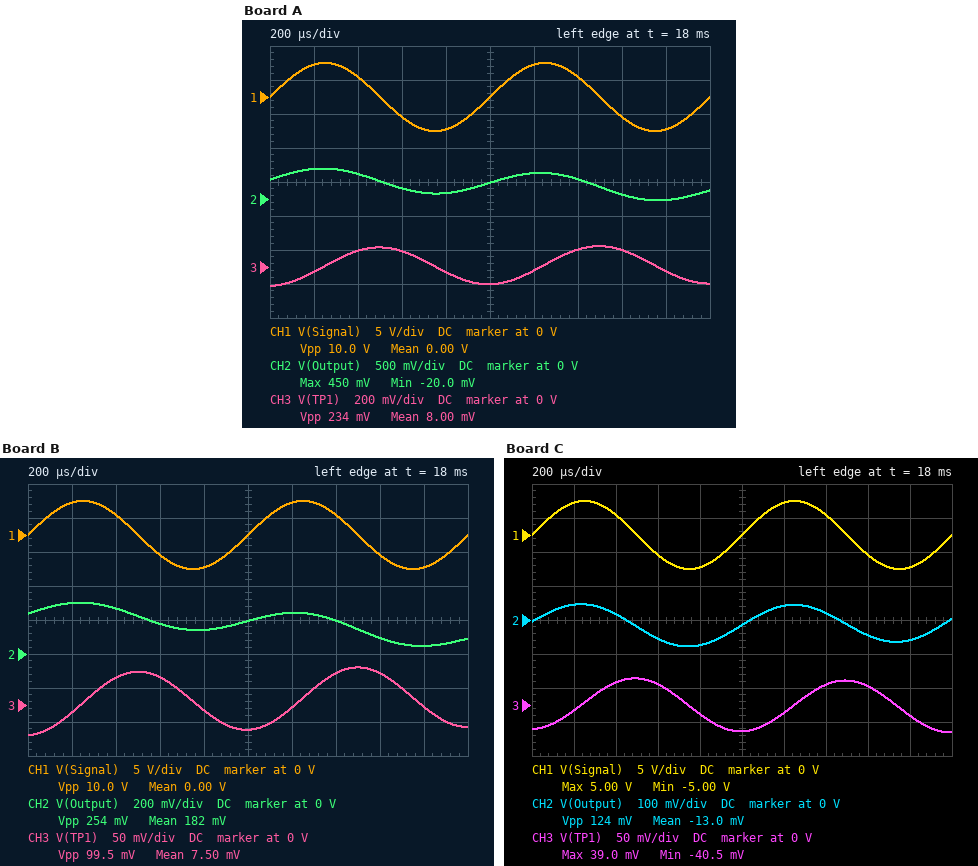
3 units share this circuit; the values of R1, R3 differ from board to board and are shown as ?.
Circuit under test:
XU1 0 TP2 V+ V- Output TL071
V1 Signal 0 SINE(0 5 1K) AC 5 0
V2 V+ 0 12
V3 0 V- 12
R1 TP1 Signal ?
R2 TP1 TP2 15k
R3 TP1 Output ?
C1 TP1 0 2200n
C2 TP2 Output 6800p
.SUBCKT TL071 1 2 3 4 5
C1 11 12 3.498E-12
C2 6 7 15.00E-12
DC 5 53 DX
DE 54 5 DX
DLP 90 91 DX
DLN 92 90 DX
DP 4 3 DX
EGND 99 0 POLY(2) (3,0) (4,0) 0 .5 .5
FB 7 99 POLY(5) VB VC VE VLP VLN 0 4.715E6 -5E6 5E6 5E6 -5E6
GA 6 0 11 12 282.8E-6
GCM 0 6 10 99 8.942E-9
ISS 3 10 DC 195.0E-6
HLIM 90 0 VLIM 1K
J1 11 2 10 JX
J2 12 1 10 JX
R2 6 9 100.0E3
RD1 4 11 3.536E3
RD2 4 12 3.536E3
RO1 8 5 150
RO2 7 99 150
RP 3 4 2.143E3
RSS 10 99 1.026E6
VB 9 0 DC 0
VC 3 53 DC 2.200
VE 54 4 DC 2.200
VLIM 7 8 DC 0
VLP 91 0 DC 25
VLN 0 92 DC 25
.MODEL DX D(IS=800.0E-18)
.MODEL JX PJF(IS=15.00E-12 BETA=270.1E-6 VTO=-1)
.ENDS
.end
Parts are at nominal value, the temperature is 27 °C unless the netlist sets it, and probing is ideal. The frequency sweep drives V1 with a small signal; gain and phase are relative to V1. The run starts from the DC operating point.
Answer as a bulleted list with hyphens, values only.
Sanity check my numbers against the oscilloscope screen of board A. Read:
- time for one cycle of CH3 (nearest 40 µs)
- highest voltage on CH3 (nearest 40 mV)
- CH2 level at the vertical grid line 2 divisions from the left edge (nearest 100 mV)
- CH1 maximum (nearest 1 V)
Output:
- 1.00 ms
- 120 mV
- 400 mV
- 5 V
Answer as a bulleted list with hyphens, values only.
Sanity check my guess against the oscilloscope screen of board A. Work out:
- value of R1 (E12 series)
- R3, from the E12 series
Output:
- 3.3 kΩ
- 12 kΩ
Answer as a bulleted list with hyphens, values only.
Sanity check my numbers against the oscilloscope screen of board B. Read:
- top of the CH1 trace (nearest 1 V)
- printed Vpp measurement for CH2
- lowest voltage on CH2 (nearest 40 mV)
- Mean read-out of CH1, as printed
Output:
- 5 V
- 254 mV
- 40 mV
- 0.00 V
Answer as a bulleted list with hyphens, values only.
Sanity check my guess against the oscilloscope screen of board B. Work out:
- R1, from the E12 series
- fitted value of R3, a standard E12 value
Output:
- 8.2 kΩ
- 12 kΩ
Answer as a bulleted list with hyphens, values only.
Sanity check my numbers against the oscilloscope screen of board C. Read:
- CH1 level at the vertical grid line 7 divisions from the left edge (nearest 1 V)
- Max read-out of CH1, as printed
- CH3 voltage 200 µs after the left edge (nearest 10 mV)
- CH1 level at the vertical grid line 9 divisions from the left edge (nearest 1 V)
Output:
- 3 V
- 5.00 V
- -10 mV
- -5 V
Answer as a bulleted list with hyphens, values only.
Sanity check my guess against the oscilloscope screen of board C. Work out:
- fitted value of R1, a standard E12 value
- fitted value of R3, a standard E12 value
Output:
- 10 kΩ
- 2.2 kΩ
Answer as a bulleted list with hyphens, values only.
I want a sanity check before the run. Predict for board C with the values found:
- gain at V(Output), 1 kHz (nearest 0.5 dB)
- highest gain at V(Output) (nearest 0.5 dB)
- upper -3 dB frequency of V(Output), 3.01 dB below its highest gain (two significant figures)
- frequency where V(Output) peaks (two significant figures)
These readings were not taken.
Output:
- -38.5 dB
- 1.0 dB
- 250 Hz
- 220 Hz
